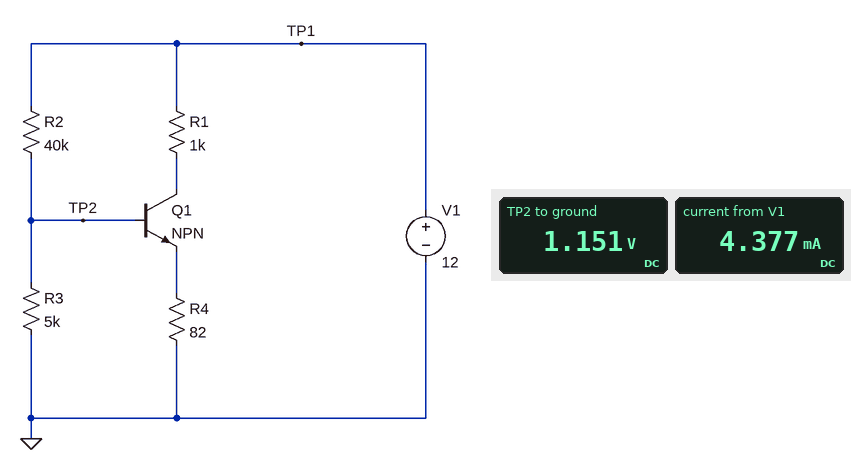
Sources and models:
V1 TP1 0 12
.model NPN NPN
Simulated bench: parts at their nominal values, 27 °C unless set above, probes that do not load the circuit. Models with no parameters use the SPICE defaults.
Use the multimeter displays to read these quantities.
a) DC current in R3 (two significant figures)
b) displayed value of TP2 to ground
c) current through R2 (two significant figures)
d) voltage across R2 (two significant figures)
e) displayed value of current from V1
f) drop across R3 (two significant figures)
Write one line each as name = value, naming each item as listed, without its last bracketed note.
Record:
DC current in R3 = 230 µA
displayed value of TP2 to ground = 1.151 V
current through R2 = 270 µA
voltage across R2 = 11 V
displayed value of current from V1 = 4.377 mA
drop across R3 = 1.2 V
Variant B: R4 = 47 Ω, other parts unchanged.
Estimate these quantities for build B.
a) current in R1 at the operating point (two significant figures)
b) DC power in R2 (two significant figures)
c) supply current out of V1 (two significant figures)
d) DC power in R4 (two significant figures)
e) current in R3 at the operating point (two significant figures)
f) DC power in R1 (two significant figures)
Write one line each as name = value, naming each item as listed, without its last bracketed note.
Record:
current in R1 at the operating point = 5.6 mA
DC power in R2 = 3.0 mW
supply current out of V1 = 5.9 mA
DC power in R4 = 1.5 mW
current in R3 at the operating point = 220 µA
DC power in R1 = 31 mW
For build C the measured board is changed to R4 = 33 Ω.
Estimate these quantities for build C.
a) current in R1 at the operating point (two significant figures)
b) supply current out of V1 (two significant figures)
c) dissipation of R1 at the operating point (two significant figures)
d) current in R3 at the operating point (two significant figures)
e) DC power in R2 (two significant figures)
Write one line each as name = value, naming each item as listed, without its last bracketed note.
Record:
current in R1 at the operating point = 6.6 mA
supply current out of V1 = 6.8 mA
dissipation of R1 at the operating point = 43 mW
current in R3 at the operating point = 210 µA
DC power in R2 = 3.0 mW
